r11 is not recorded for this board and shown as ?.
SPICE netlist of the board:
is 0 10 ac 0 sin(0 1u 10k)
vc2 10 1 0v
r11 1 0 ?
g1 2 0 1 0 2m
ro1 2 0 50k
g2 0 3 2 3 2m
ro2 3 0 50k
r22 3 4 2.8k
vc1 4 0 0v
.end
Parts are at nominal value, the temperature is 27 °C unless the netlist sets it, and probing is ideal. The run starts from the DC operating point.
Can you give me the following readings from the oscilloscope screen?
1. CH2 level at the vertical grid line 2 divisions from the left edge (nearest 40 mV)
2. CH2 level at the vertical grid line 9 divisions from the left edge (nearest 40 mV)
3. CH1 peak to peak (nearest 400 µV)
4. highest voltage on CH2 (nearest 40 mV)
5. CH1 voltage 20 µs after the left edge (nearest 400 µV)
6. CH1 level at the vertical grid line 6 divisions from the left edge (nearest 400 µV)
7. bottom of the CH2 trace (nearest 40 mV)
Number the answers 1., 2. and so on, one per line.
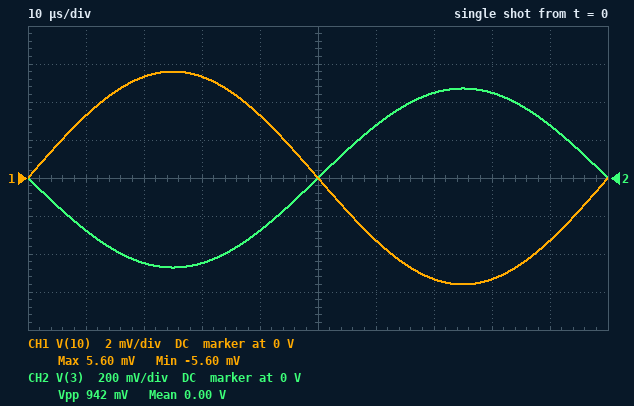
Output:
1. -440 mV
2. 280 mV
3. 11.2 mV
4. 480 mV
5. 5.2 mV
6. -3.2 mV
7. -480 mV
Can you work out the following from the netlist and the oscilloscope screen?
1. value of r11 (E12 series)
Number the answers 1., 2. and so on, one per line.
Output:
1. 5.6 kΩ
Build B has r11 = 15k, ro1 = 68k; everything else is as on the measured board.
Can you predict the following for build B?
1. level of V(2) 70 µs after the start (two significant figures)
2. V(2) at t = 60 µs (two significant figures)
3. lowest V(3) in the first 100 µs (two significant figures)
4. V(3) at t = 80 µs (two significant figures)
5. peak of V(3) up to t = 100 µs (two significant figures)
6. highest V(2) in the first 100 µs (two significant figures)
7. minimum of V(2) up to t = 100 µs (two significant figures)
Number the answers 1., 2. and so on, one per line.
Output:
1. 1.9 V
2. 1.2 V
3. -1.7 V
4. 1.6 V
5. 1.7 V
6. 2.0 V
7. -2.0 V
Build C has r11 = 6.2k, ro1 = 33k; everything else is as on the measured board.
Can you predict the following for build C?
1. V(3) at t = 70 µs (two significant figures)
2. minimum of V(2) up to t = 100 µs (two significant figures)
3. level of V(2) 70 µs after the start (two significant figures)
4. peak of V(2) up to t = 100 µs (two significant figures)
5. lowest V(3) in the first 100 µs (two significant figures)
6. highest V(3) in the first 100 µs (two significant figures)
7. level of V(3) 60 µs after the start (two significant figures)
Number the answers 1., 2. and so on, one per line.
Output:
1. 330 mV
2. -410 mV
3. 390 mV
4. 410 mV
5. -340 mV
6. 340 mV
7. 200 mV
